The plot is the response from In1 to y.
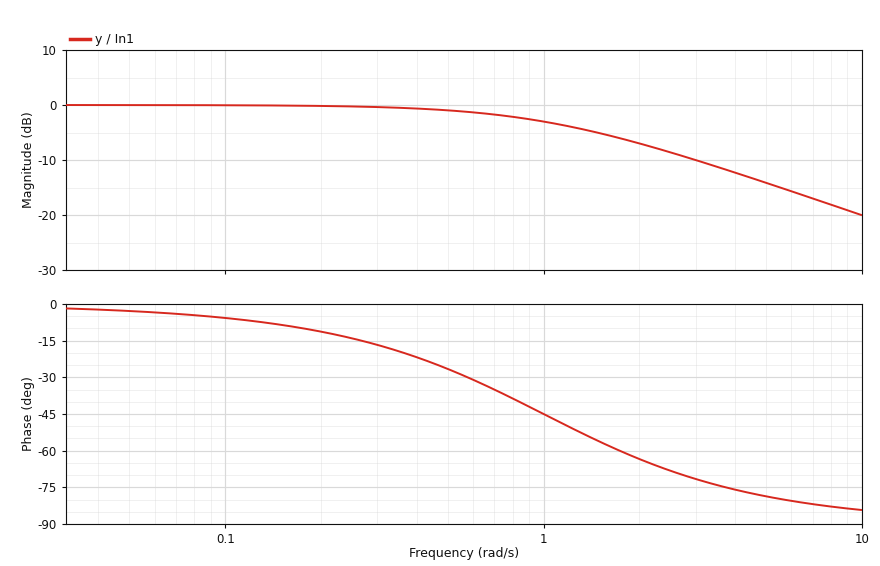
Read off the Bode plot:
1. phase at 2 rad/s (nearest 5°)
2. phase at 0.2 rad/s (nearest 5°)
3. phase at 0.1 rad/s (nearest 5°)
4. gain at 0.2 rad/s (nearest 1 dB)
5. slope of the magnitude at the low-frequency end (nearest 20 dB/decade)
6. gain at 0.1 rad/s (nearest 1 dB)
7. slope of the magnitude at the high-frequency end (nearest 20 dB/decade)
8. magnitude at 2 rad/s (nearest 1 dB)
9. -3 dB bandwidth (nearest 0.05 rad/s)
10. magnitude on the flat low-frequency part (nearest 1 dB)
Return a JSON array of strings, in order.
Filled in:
["-65°", "-10°", "-5°", "0 dB", "0 dB/decade", "0 dB", "-20 dB/decade", "-7 dB", "1.00 rad/s", "0 dB"]
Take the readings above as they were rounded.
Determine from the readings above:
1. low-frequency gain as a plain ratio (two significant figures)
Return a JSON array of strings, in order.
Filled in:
["1.0"]
